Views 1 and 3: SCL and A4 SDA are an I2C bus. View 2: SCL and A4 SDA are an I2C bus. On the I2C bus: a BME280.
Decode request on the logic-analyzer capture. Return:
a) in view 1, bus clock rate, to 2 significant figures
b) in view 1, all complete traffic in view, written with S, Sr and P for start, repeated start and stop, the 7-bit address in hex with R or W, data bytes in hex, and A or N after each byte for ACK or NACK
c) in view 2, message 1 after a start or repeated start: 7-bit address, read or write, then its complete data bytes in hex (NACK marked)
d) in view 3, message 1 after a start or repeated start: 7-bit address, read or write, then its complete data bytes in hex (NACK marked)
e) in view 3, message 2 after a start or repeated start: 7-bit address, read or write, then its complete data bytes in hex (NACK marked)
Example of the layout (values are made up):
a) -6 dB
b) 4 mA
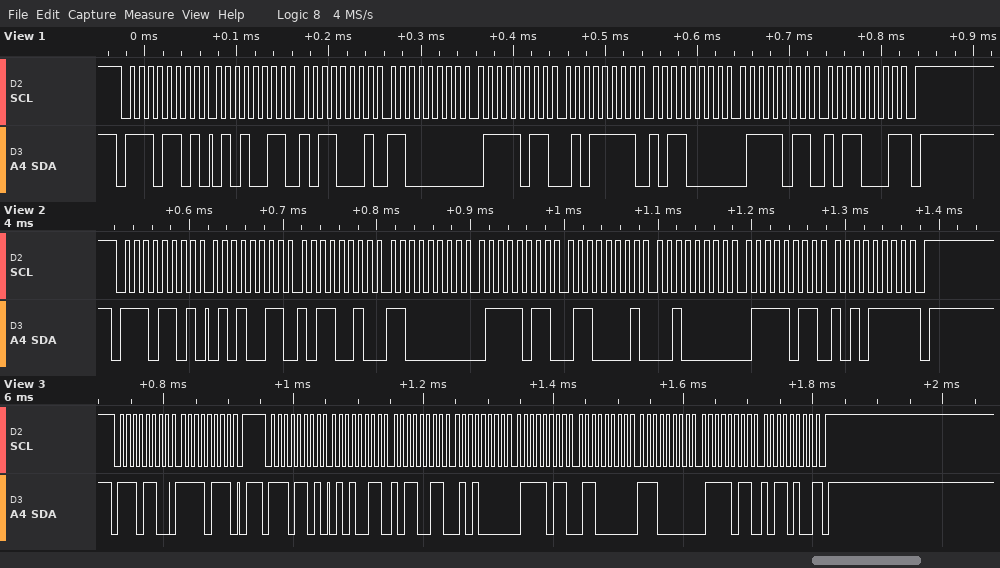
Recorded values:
a) 100 kHz
b) S 76R A 53 A B1 A C0 A 7B A 5F A B0 A 7B A B1 N P
c) 0x76 read: 53 B2 C0 7B 61 20 7B AF NACK
d) 0x76 write: F7
e) 0x76 read: 53 B3 50 7B 60 E0 7B B4 NACK
